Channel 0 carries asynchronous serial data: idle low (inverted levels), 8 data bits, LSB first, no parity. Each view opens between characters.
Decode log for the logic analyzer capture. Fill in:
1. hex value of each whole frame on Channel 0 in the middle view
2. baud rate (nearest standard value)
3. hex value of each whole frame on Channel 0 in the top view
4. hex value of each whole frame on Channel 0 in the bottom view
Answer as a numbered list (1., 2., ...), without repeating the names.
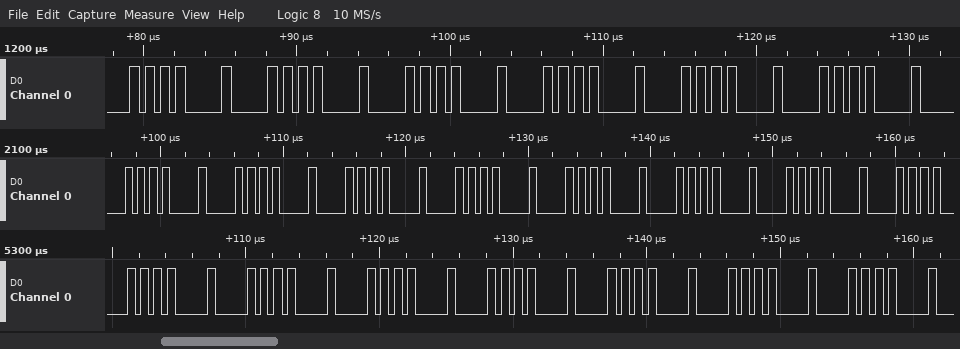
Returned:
1. D5, 5F, 7D, D5, 5F, 7D, D5, 5F, 7D, D5, 5F
2. 2000000 baud
3. D5, 5F, 7D, D5, 5F, 7D, D5, 5F, 7D
4. D5, 5F, 7D, D5, 5F, 7D, D5, 5F, 7D, D5
